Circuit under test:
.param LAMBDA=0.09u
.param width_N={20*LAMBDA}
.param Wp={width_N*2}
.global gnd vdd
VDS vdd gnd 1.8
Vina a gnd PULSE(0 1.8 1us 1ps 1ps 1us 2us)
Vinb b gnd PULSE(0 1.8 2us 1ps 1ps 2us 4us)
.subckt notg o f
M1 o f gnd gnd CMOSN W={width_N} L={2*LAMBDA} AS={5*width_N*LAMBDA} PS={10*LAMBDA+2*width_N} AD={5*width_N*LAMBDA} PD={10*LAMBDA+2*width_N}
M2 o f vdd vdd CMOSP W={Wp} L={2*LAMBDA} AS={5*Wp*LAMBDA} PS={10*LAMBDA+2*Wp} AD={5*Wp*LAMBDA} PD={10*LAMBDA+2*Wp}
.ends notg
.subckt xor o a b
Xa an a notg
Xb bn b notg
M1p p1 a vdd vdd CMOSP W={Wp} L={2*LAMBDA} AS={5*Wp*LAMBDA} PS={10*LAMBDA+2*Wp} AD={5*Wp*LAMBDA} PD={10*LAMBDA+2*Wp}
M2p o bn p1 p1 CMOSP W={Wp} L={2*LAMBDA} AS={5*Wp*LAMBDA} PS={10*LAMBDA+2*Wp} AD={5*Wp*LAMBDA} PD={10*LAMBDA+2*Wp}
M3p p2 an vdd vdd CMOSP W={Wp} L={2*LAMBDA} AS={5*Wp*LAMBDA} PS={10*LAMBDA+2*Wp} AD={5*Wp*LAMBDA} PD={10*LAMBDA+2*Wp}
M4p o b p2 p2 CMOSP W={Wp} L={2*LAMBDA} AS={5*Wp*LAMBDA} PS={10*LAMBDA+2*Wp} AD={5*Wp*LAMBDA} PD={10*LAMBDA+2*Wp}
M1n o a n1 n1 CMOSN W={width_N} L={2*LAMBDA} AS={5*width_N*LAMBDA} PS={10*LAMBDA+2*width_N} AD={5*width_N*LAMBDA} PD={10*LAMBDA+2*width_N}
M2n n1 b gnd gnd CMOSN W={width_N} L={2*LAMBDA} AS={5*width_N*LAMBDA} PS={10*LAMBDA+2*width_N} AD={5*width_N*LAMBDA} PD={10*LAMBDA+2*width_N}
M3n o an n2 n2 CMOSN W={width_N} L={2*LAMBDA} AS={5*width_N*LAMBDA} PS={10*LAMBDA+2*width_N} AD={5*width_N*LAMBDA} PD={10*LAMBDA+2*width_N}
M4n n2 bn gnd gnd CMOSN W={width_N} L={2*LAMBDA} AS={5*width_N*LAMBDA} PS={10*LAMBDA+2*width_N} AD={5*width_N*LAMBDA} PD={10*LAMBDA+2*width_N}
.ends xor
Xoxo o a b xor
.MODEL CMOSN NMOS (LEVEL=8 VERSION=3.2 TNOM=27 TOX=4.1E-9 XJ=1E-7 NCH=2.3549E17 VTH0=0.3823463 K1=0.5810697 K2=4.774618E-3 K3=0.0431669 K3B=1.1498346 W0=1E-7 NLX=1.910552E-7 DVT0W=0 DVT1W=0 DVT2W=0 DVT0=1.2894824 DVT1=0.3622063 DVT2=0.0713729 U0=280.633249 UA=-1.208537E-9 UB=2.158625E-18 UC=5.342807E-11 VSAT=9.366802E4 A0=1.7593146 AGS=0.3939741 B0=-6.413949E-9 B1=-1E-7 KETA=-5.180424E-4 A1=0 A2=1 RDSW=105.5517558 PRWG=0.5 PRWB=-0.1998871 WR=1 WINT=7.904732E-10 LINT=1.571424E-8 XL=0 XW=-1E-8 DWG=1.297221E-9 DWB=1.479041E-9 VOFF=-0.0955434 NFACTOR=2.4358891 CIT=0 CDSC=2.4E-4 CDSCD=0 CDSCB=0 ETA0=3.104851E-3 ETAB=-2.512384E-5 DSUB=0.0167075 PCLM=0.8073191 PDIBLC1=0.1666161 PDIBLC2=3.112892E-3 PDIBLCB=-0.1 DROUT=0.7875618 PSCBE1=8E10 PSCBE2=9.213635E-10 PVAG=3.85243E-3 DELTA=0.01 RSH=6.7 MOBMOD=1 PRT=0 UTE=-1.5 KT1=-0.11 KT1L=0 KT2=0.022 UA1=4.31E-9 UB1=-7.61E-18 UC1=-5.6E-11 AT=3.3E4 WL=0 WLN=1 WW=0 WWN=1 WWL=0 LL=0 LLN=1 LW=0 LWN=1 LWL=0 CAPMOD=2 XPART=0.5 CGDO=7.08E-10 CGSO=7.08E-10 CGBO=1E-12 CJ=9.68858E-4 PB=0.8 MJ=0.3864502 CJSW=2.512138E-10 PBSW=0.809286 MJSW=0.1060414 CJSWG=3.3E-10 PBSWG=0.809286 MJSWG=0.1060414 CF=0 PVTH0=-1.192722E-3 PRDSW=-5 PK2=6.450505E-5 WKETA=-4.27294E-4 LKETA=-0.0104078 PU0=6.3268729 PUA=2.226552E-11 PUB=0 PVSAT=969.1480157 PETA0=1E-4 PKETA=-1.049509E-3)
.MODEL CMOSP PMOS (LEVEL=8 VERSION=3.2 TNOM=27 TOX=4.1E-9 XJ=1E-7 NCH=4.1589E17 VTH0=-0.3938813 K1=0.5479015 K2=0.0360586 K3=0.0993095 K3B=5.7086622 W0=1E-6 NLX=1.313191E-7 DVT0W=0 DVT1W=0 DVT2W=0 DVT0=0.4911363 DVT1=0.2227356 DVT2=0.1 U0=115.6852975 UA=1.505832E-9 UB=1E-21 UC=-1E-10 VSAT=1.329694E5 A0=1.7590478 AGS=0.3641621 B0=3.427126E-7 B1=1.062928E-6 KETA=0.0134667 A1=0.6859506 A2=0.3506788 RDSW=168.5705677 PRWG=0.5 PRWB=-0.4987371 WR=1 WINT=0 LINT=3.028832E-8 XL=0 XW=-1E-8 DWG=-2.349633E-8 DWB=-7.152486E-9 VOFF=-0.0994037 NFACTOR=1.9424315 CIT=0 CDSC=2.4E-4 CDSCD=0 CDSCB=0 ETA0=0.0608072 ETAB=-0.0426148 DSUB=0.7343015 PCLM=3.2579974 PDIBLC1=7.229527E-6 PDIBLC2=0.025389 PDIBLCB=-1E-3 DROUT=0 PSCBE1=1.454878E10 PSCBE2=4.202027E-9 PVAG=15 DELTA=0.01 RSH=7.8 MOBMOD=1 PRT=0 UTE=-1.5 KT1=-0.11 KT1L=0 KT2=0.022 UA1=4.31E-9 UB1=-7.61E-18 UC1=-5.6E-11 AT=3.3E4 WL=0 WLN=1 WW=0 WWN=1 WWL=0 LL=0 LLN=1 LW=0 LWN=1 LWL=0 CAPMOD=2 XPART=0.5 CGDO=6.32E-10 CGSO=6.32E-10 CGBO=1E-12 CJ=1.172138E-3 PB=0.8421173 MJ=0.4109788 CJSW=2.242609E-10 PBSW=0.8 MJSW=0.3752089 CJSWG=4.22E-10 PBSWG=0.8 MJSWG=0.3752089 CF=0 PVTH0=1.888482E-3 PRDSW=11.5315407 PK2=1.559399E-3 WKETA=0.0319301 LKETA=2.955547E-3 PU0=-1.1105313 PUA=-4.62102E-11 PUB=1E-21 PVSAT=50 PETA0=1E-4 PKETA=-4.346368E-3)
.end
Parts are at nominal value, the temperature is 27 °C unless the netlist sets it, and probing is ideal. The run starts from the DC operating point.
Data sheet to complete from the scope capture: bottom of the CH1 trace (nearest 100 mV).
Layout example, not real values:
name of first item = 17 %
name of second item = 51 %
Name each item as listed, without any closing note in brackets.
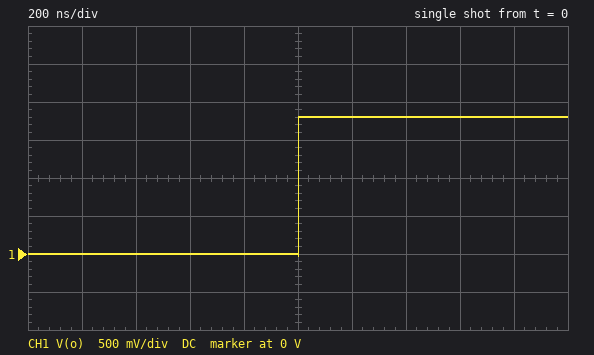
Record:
bottom of the CH1 trace = 0 V
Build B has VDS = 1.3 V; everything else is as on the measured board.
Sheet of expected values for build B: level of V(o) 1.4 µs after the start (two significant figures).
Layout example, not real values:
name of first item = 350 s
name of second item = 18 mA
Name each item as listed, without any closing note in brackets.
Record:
level of V(o) 1.4 µs after the start = 1.3 V
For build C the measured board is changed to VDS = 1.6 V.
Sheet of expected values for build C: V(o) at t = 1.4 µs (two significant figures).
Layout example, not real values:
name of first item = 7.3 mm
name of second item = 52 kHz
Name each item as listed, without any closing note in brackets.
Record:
V(o) at t = 1.4 µs = 1.6 V
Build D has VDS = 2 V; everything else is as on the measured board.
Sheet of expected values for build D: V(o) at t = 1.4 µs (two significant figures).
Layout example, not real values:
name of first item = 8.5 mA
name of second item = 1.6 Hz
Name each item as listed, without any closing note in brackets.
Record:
V(o) at t = 1.4 µs = 2.0 V
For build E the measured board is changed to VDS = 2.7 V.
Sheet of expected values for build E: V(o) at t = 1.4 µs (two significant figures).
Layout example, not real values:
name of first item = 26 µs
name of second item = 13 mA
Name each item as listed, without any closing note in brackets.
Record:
V(o) at t = 1.4 µs = 2.7 V
